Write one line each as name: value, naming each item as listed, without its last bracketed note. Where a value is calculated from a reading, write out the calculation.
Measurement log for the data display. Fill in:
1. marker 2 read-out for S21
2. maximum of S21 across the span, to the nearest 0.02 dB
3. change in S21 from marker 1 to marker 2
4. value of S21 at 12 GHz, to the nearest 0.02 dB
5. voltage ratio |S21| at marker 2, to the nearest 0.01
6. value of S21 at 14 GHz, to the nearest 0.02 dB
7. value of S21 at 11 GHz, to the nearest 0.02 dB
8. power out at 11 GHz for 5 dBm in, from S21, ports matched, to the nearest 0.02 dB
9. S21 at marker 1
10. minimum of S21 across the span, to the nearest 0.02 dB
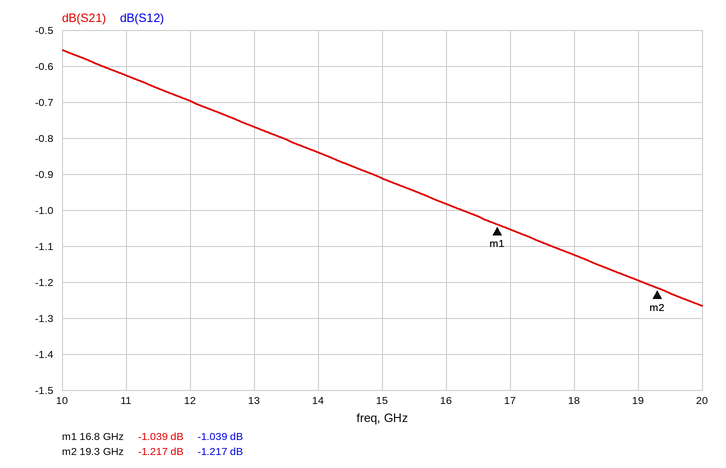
marker 2 read-out for S21: -1.217 dB
maximum of S21 across the span, to the nearest 0.02 dB: -0.56 dB
change in S21 from marker 1 to marker 2: -1.217 − (-1.039) = -0.178 dB
value of S21 at 12 GHz, to the nearest 0.02 dB: -0.70 dB
voltage ratio |S21| at marker 2, to the nearest 0.01: 10^(-1.217/20) ≈ 0.87
value of S21 at 14 GHz, to the nearest 0.02 dB: -0.84 dB
value of S21 at 11 GHz, to the nearest 0.02 dB: -0.62 dB
power out at 11 GHz for 5 dBm in, from S21, ports matched, to the nearest 0.02 dB: 5 dBm + (-0.62 dB) = 4.38 dBm
S21 at marker 1: -1.039 dB
minimum of S21 across the span, to the nearest 0.02 dB: -1.26 dB
